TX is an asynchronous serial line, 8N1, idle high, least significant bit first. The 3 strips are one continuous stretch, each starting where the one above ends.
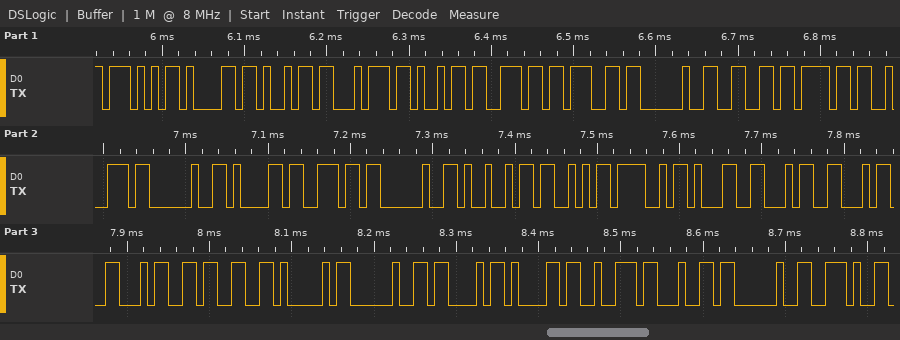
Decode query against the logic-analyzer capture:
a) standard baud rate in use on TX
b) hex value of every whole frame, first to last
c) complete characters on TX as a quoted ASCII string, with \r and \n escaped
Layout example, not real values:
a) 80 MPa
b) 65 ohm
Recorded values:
a) 115200 baud
b) 0x57 0x61 0x69 0x74 0x69 0x6E 0x67 0x20 0x66 0x6F 0x72 0x20 0x61 0x6E 0x20 0x49 0x53 0x4F 0x31 0x34 0x34 0x34 0x33 0x41 0x20 0x43 0x61 0x72 0x64 0x20 0x2E
c) "Waiting for an ISO14443A Card ."
